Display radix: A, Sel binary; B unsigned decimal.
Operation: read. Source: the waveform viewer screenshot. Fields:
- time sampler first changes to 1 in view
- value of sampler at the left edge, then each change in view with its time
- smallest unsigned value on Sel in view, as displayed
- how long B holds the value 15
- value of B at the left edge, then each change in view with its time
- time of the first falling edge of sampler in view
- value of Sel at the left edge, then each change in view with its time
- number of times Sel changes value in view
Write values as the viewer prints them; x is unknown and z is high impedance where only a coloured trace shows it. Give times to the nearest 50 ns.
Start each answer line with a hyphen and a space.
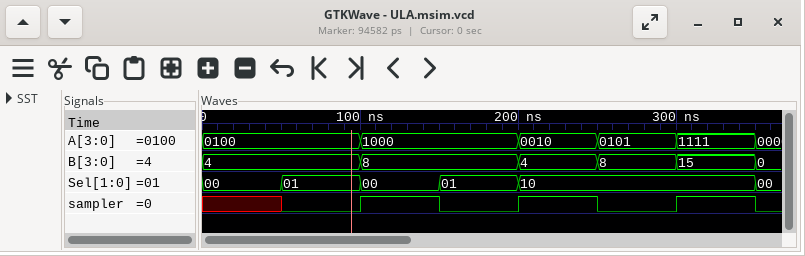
- 100 ns
- x, 0 at 50 ns, 1 at 100 ns, 0 at 150 ns, 1 at 200 ns, 0 at 250 ns, 1 at 300 ns, 0 at 350 ns
- 00
- 50 ns
- 4, 8 at 100 ns, 4 at 200 ns, 8 at 250 ns, 15 at 300 ns, 0 at 350 ns
- 150 ns
- 00, 01 at 50 ns, 00 at 100 ns, 01 at 150 ns, 10 at 200 ns, 00 at 350 ns
- 5
